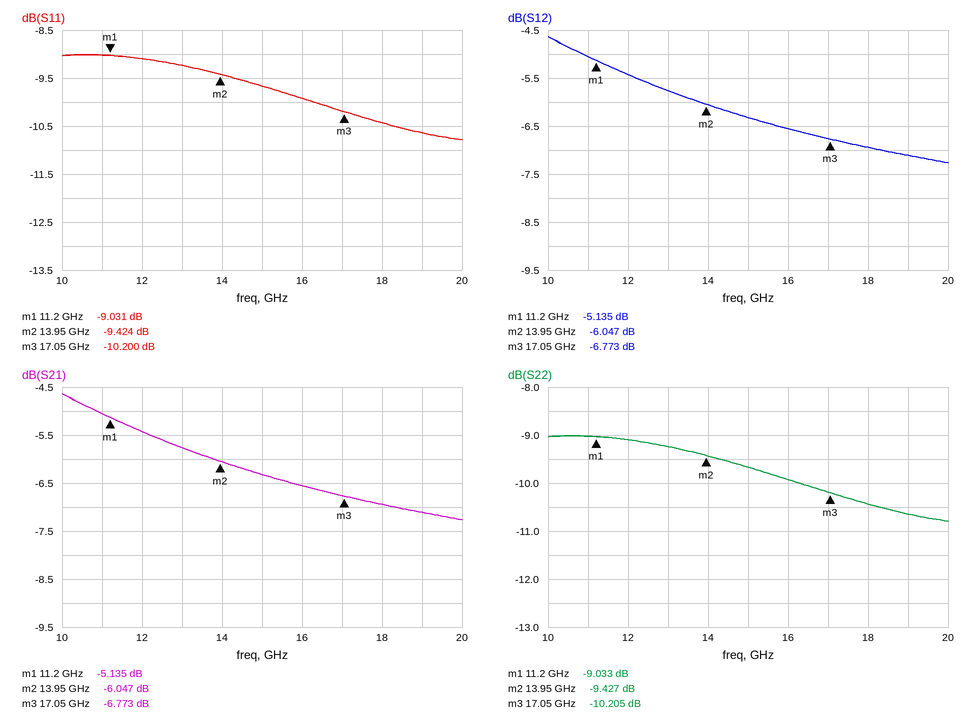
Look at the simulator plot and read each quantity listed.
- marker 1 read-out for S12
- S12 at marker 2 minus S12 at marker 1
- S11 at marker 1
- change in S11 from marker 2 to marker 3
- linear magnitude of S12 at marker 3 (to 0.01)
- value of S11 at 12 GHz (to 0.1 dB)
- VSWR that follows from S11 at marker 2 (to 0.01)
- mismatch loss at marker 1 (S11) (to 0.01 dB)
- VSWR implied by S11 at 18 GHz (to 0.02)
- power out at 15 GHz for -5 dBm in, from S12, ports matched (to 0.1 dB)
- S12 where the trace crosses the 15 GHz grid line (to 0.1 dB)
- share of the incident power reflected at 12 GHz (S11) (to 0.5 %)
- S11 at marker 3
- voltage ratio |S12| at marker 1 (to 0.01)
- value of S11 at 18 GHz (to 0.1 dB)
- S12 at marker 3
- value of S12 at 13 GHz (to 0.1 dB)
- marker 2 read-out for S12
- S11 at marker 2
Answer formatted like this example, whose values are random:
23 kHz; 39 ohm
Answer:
-5.135 dB; -0.912 dB; -9.031 dB; -0.776 dB; 0.46; -9.1 dB; 2.02; 0.58 dB; 1.86; -11.3 dBm; -6.3 dB; 12.5 %; -10.200 dB; 0.55; -10.4 dB; -6.773 dB; -5.8 dB; -6.047 dB; -9.424 dB
